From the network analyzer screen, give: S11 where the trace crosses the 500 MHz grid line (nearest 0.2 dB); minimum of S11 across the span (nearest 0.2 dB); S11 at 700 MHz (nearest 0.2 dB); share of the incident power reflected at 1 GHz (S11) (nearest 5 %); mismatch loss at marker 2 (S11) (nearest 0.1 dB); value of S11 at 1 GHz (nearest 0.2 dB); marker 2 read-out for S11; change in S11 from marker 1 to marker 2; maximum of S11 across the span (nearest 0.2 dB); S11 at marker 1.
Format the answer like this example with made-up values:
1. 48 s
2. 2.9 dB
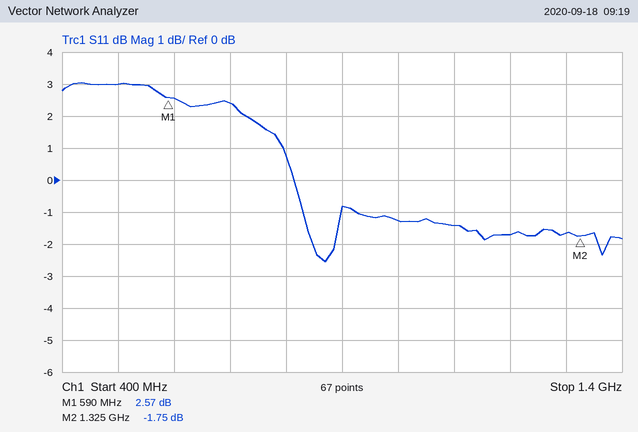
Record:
1. 3.0 dB
2. -2.6 dB
3. 2.4 dB
4. 75 %
5. 4.8 dB
6. -1.2 dB
7. -1.75 dB
8. -4.32 dB
9. 3.0 dB
10. 2.57 dB
